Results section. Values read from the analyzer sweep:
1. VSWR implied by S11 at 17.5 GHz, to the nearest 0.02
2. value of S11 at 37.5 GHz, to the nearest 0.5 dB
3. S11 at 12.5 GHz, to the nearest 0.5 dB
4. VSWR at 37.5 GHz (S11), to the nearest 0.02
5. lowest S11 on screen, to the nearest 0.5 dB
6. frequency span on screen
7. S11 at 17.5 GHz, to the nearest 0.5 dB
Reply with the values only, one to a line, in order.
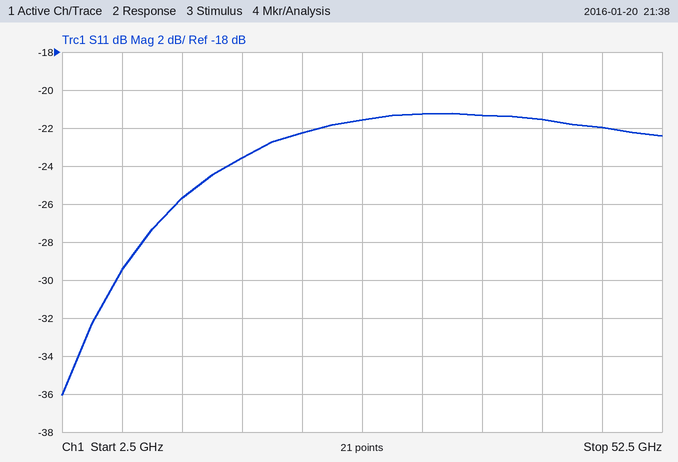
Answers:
1.14
-21.5 dB
-25.5 dB
1.18
-36.0 dB
50 GHz
-23.5 dB
